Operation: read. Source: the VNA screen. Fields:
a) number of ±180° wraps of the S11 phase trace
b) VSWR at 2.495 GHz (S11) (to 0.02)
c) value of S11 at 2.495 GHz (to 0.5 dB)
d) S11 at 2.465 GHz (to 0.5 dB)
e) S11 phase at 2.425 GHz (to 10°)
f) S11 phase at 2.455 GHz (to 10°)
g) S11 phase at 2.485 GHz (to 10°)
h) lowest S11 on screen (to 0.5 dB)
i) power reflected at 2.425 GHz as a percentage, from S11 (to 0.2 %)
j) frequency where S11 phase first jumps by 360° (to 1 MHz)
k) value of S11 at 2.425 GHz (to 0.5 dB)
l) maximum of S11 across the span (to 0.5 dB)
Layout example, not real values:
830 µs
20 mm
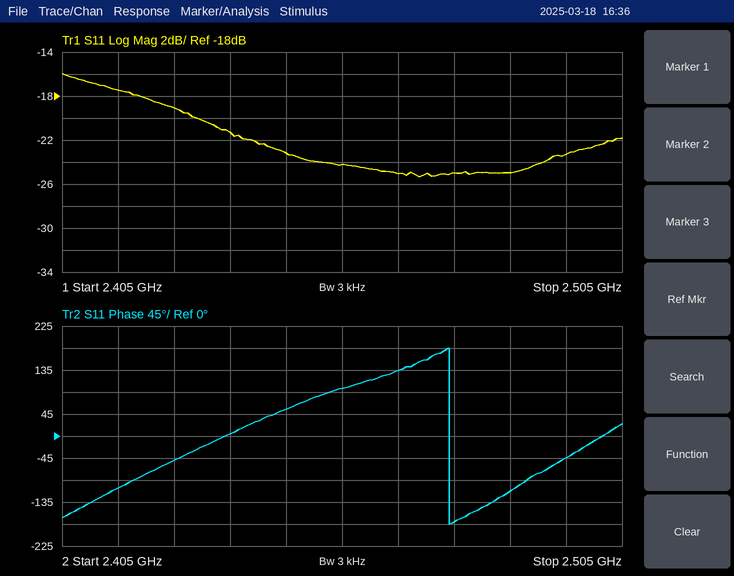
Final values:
1
1.14
-23.5 dB
-25.0 dB
-50°
100°
-110°
-25.5 dB
1.2 %
2.474 GHz
-19.0 dB
-16.0 dB
